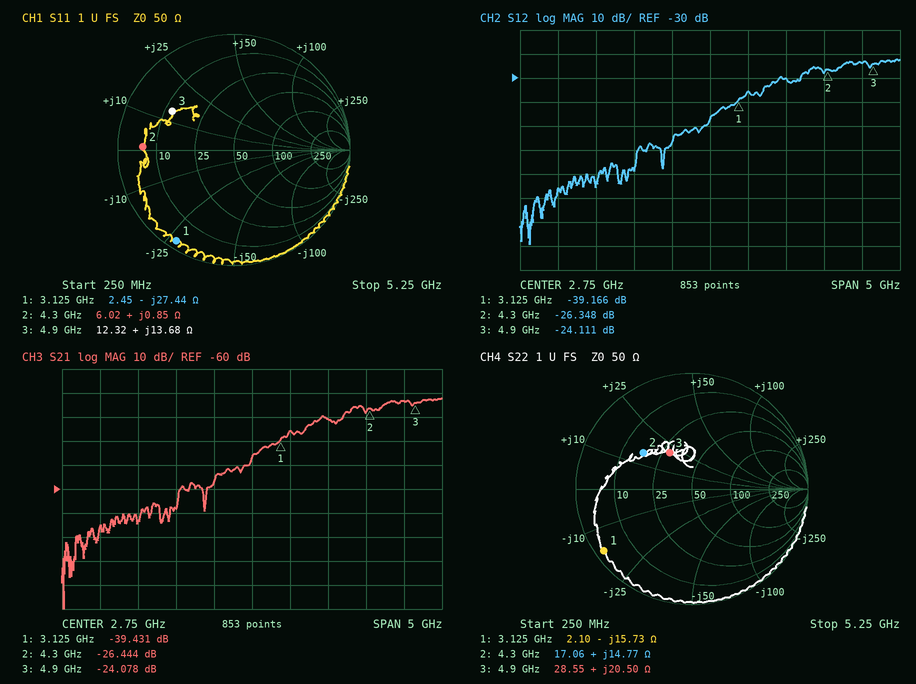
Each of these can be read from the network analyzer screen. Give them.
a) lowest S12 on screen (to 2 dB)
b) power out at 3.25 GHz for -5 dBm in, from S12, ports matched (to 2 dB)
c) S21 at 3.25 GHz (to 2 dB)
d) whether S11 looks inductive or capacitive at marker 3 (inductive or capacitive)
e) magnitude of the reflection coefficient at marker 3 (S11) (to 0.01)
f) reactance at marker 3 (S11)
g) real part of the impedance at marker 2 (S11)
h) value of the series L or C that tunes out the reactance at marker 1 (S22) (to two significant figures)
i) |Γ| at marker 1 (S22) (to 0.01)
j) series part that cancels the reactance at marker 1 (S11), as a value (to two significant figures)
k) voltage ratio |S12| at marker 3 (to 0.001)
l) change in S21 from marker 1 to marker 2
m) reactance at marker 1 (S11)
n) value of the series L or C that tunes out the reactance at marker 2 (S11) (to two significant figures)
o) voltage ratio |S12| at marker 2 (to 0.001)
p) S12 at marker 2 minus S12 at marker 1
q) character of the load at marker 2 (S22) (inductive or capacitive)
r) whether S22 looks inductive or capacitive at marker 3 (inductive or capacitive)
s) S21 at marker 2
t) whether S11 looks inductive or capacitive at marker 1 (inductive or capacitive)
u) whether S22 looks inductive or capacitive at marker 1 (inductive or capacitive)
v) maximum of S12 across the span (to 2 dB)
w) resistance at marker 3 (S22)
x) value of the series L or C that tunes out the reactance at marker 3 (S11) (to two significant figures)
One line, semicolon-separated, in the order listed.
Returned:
-100 dB; -40 dBm; -36 dB; inductive; 0.63; +13.68 Ω; 6.02 Ω; 800 pH; 0.93; 1.4 nH; 0.062; 12.987 dB; -27.44 Ω; 44 pF; 0.048; 12.818 dB; inductive; inductive; -26.444 dB; capacitive; capacitive; -22 dB; 28.55 Ω; 2.4 pF
